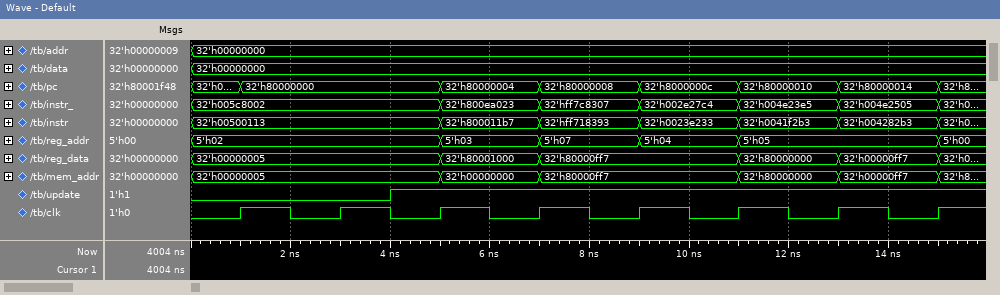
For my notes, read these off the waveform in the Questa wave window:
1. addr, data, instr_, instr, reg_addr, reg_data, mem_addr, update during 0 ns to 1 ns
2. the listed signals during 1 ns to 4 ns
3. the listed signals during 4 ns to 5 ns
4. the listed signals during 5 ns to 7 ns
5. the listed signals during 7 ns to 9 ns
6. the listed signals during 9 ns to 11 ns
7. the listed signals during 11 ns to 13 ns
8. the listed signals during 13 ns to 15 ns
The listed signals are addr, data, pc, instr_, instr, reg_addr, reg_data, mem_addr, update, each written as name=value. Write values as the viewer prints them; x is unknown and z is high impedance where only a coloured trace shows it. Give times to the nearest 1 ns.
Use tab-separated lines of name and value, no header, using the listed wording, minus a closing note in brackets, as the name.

addr, data, instr_, instr, reg_addr, reg_data, mem_addr, update during 0 ns to 1 ns	addr=32'h00000000, data=32'h00000000, instr_=32'h005c8002, instr=32'h00500113, reg_addr=5'h02, reg_data=32'h00000005, mem_addr=32'h00000005, update=0
the listed signals during 1 ns to 4 ns	addr=32'h00000000, data=32'h00000000, pc=32'h80000000, instr_=32'h005c8002, instr=32'h00500113, reg_addr=5'h02, reg_data=32'h00000005, mem_addr=32'h00000005, update=0
the listed signals during 4 ns to 5 ns	addr=32'h00000000, data=32'h00000000, pc=32'h80000000, instr_=32'h005c8002, instr=32'h00500113, reg_addr=5'h02, reg_data=32'h00000005, mem_addr=32'h00000005, update=1
the listed signals during 5 ns to 7 ns	addr=32'h00000000, data=32'h00000000, pc=32'h80000004, instr_=32'h800ea023, instr=32'h800011b7, reg_addr=5'h03, reg_data=32'h80001000, mem_addr=32'h00000000, update=1
the listed signals during 7 ns to 9 ns	addr=32'h00000000, data=32'h00000000, pc=32'h80000008, instr_=32'hff7c8307, instr=32'hff718393, reg_addr=5'h07, reg_data=32'h80000ff7, mem_addr=32'h80000ff7, update=1
the listed signals during 9 ns to 11 ns	addr=32'h00000000, data=32'h00000000, pc=32'h8000000c, instr_=32'h002e27c4, instr=32'h0023e233, reg_addr=5'h04, reg_data=32'h80000ff7, mem_addr=32'h80000ff7, update=1
the listed signals during 11 ns to 13 ns	addr=32'h00000000, data=32'h00000000, pc=32'h80000010, instr_=32'h004e23e5, instr=32'h0041f2b3, reg_addr=5'h05, reg_data=32'h80000000, mem_addr=32'h80000000, update=1
the listed signals during 13 ns to 15 ns	addr=32'h00000000, data=32'h00000000, pc=32'h80000014, instr_=32'h004e2505, instr=32'h004282b3, reg_addr=5'h05, reg_data=32'h00000ff7, mem_addr=32'h00000ff7, update=1
